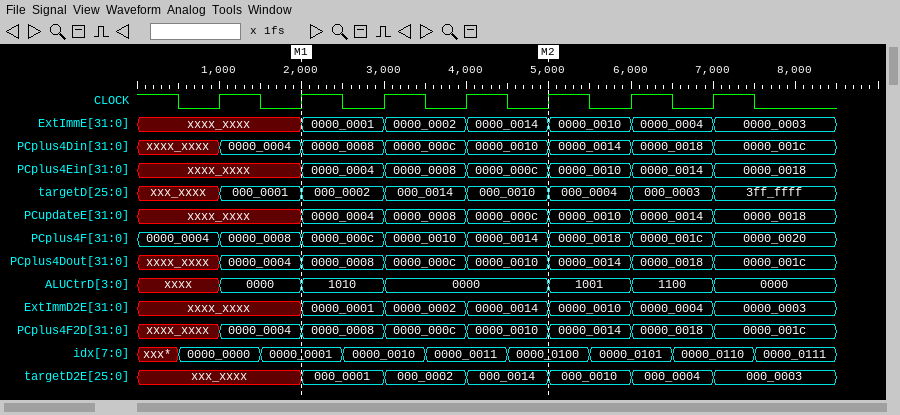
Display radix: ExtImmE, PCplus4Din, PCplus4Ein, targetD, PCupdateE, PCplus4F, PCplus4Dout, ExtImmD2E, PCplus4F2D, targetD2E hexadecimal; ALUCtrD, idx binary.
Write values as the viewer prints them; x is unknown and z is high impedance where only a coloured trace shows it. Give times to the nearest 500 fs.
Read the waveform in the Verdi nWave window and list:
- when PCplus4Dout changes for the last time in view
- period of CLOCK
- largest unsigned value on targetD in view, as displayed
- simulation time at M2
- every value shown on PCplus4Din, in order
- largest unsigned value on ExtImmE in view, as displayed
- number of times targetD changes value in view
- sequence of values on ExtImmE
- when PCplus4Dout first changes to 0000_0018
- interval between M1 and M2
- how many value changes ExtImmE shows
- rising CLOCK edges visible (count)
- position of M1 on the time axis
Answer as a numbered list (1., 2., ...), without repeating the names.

1. 7000 fs
2. 1000 fs
3. 3ff_ffff
4. 5000 fs
5. xxxx_xxxx, 0000_0004, 0000_0008, 0000_000c, 0000_0010, 0000_0014, 0000_0018, 0000_001c
6. 0000_0014
7. 7
8. xxxx_xxxx, 0000_0001, 0000_0002, 0000_0014, 0000_0010, 0000_0004, 0000_0003
9. 6000 fs
10. 3000 fs
11. 6
12. 7
13. 2000 fs
